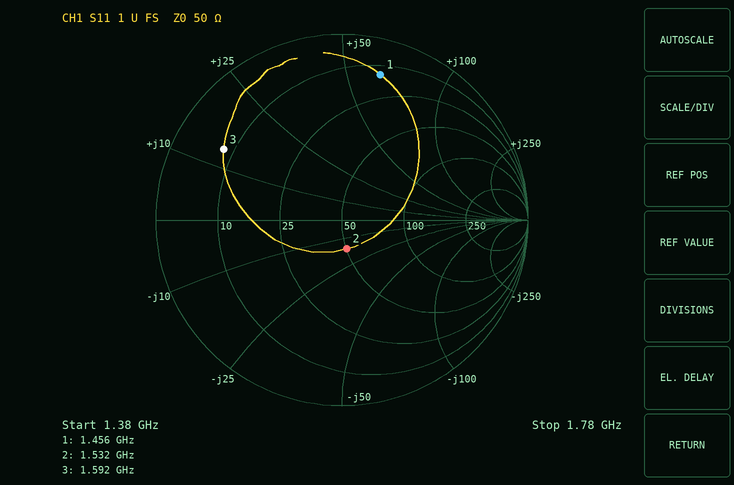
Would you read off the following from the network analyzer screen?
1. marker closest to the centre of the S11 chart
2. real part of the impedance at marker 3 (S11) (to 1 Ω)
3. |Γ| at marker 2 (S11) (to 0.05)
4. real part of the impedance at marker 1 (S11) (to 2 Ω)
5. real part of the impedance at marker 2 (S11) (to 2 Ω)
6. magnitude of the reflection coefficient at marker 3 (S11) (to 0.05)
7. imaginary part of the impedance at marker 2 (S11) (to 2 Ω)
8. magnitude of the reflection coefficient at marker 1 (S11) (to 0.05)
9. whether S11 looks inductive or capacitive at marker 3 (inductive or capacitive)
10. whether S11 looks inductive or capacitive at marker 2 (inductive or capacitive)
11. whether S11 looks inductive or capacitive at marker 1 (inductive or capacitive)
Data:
marker 2
8 Ω
0.15
14 Ω
50 Ω
0.75
-16 Ω
0.80
inductive
capacitive
inductive
